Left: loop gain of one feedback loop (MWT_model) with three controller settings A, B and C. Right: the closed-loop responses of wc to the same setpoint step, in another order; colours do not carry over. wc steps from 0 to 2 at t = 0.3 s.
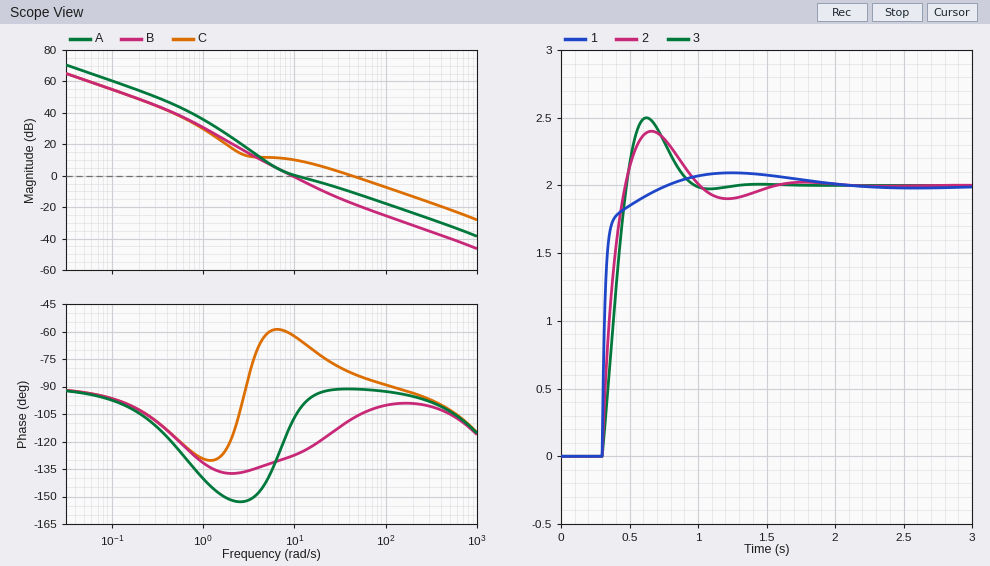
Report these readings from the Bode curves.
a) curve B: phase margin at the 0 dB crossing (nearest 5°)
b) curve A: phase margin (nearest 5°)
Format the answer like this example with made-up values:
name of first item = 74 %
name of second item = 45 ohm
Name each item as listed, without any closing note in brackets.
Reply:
curve B: phase margin at the 0 dB crossing = 50°
curve A: phase margin = 75°
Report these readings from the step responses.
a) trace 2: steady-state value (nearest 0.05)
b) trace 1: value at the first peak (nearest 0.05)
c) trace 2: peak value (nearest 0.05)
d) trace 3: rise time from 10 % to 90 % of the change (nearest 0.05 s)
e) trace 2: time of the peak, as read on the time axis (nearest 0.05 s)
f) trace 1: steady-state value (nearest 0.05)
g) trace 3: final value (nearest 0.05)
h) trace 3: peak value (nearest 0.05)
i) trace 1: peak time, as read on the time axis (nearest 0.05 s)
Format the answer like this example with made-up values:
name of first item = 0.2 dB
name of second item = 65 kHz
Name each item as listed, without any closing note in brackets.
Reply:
trace 2: steady-state value = 2.00
trace 1: value at the first peak = 2.10
trace 2: peak value = 2.40
trace 3: rise time from 10 % to 90 % of the change = 0.15 s
trace 2: time of the peak, as read on the time axis = 0.65 s
trace 1: steady-state value = 2.00
trace 3: final value = 2.00
trace 3: peak value = 2.50
trace 1: peak time, as read on the time axis = 1.25 s
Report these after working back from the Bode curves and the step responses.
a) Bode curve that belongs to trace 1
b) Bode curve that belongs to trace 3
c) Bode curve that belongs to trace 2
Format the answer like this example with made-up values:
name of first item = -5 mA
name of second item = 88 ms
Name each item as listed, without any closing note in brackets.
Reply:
Bode curve that belongs to trace 1 = C
Bode curve that belongs to trace 3 = B
Bode curve that belongs to trace 2 = A
